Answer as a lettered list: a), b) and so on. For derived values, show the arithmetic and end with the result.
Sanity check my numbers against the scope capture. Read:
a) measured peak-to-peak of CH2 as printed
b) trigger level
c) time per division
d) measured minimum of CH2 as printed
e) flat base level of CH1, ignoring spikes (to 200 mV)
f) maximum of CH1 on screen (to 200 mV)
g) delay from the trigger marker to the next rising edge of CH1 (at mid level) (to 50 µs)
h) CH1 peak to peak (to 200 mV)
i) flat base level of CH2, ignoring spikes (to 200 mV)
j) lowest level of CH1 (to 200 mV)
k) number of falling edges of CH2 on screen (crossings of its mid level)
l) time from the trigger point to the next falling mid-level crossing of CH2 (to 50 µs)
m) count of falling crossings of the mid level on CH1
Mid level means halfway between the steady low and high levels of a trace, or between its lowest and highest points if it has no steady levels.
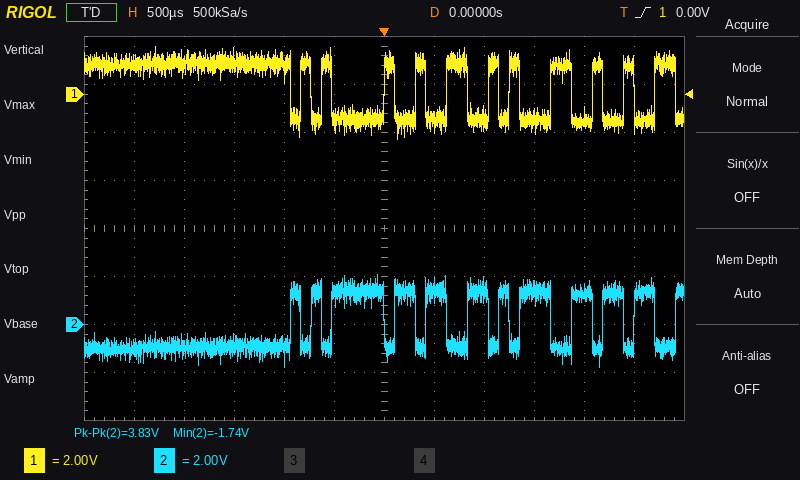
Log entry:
a) 3.83 V
b) 0.00 V
c) 500 µs
d) -1.74 V
e) -1.0 V
f) 2.0 V
g) 300 µs
h) 2.0 V − (-1.8 V) = 3.8 V
i) -1.0 V
j) -1.8 V
k) 11
l) 300 µs
m) 12
